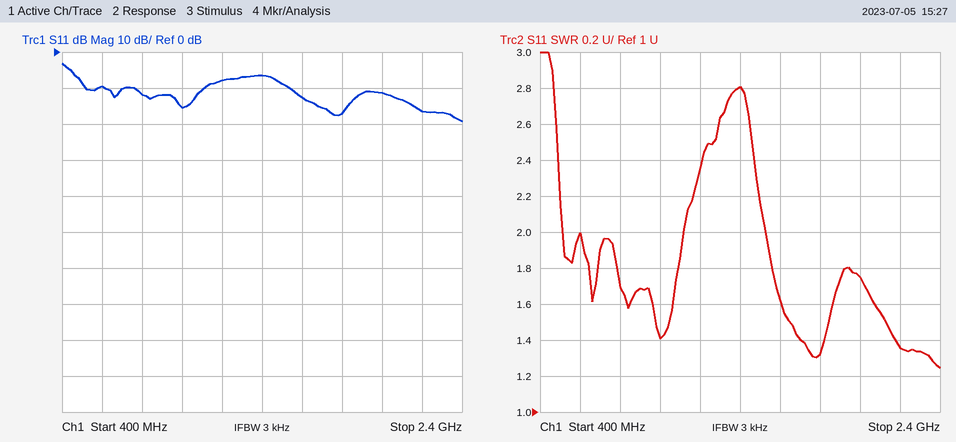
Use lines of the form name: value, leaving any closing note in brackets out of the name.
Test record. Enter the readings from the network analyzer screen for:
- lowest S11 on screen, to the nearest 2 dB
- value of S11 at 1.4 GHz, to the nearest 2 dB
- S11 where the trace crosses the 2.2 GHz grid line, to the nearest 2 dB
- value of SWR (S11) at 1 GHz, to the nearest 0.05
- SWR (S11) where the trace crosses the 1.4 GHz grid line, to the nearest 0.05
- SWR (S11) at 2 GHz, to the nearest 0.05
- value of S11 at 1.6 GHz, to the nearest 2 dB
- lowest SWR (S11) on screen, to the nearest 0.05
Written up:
lowest S11 on screen, to the nearest 2 dB: -20 dB
value of S11 at 1.4 GHz, to the nearest 2 dB: -6 dB
S11 where the trace crosses the 2.2 GHz grid line, to the nearest 2 dB: -16 dB
value of SWR (S11) at 1 GHz, to the nearest 0.05: 1.40
SWR (S11) where the trace crosses the 1.4 GHz grid line, to the nearest 0.05: 2.80
SWR (S11) at 2 GHz, to the nearest 0.05: 1.75
value of S11 at 1.6 GHz, to the nearest 2 dB: -12 dB
lowest SWR (S11) on screen, to the nearest 0.05: 1.25
